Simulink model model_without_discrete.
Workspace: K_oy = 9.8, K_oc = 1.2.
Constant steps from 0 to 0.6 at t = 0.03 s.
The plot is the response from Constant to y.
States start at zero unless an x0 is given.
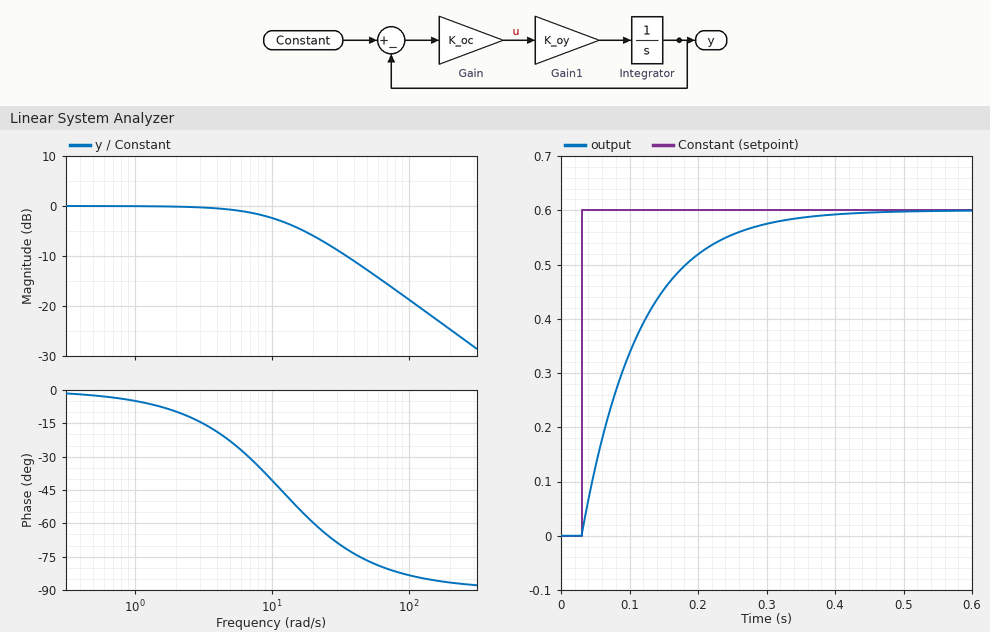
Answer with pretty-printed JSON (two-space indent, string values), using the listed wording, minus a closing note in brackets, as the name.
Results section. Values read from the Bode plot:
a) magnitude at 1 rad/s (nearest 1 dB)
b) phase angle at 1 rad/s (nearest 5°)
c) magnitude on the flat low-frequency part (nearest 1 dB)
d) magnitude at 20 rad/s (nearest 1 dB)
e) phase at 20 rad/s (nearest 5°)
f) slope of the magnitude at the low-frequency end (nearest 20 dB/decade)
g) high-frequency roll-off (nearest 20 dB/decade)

{
  "magnitude at 1 rad/s": "0 dB",
  "phase angle at 1 rad/s": "-5°",
  "magnitude on the flat low-frequency part": "0 dB",
  "magnitude at 20 rad/s": "-6 dB",
  "phase at 20 rad/s": "-60°",
  "slope of the magnitude at the low-frequency end": "0 dB/decade",
  "high-frequency roll-off": "-20 dB/decade"
}
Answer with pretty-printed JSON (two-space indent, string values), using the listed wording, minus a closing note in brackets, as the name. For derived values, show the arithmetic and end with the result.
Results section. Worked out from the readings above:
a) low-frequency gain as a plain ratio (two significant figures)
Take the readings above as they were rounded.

{
  "low-frequency gain as a plain ratio": "10^(0 / 20) = 1.0"
}
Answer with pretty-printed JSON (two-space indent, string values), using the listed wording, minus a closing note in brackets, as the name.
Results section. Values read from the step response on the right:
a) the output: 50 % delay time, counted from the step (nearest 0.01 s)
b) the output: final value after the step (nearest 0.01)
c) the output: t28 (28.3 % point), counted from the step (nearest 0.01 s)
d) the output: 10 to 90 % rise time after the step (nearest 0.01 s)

{
  "the output: 50 % delay time, counted from the step": "0.06 s",
  "the output: final value after the step": "0.60",
  "the output: t28 (28.3 % point), counted from the step": "0.03 s",
  "the output: 10 to 90 % rise time after the step": "0.19 s"
}
